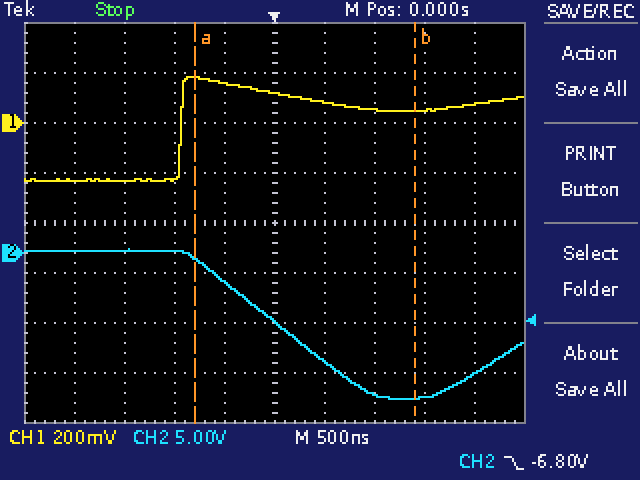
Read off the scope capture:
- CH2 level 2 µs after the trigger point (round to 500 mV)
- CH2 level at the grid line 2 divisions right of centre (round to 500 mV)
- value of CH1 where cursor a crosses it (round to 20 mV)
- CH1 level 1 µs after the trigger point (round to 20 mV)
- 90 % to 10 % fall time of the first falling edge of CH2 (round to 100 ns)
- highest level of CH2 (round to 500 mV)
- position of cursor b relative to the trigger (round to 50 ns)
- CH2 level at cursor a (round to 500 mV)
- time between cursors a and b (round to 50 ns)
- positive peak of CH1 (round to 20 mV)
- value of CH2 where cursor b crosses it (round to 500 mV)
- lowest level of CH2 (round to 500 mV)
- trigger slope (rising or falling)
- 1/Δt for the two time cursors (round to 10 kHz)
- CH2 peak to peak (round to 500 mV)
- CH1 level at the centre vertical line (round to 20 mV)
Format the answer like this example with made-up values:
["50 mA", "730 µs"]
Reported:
["-12.0 V", "-14.0 V", "180 mV", "60 mV", "1.5 µs", "500 mV", "+1.40 µs", "-500 mV", "2.20 µs", "180 mV", "-14.5 V", "-14.5 V", "falling", "450 kHz", "15.0 V", "120 mV"]
